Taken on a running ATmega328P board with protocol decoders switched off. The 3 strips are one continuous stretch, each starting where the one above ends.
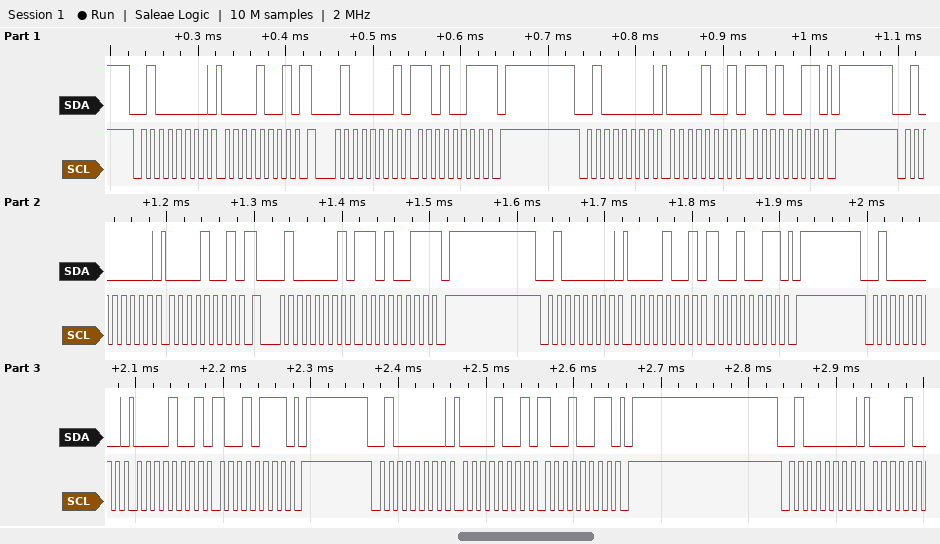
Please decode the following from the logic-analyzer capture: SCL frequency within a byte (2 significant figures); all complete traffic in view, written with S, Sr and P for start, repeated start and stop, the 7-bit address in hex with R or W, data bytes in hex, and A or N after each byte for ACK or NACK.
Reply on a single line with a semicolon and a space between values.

100 kHz; S 20W A 09 A Sr 20R A D3 N P S 20W A 09 A D3 A P S 20W A 09 A Sr 20R A D3 N P S 20W A 09 A 93 A P S 20W A 09 A 97 A P S 20W A 09 A 93 A P S 20W A
